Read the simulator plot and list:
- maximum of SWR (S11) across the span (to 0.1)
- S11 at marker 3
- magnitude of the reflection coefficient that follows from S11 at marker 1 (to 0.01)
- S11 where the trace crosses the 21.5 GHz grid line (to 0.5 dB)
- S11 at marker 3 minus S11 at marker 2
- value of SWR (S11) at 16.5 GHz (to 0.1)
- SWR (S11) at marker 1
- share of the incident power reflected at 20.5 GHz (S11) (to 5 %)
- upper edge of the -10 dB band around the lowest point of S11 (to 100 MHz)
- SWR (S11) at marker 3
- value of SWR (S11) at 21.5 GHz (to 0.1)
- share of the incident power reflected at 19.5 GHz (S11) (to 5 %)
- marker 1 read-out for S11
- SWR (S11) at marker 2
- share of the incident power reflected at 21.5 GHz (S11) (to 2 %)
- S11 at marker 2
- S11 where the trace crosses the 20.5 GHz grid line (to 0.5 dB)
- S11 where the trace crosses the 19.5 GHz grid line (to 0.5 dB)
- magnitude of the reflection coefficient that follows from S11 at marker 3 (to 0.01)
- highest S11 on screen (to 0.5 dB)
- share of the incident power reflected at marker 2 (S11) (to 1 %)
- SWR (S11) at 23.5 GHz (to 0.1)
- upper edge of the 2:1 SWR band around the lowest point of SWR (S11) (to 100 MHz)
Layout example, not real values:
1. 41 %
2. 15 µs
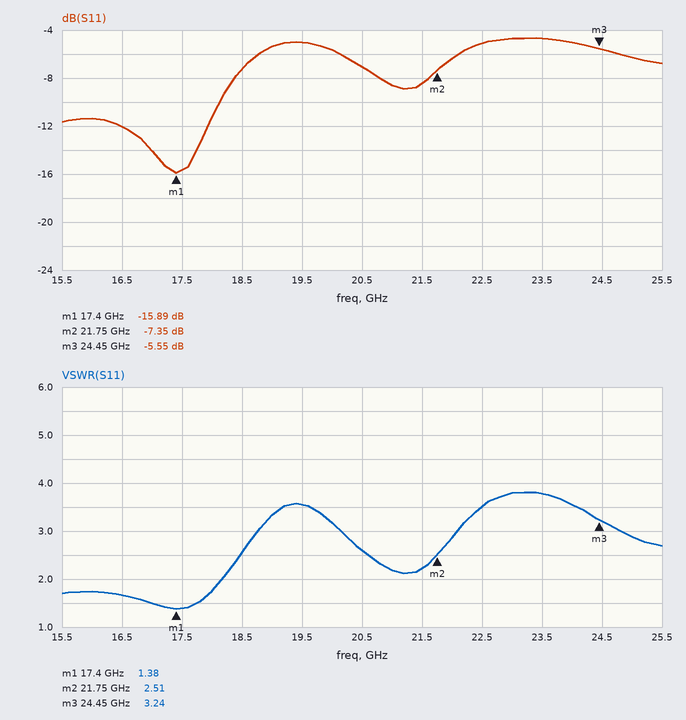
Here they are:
1. 3.8
2. -5.55 dB
3. 0.16
4. -8.5 dB
5. 1.80 dB
6. 1.7
7. 1.38
8. 20 %
9. 18.1 GHz
10. 3.24
11. 2.2
12. 30 %
13. -15.89 dB
14. 2.51
15. 14 %
16. -7.35 dB
17. -7.0 dB
18. -5.0 dB
19. 0.53
20. -4.5 dB
21. 18 %
22. 3.8
23. 18.2 GHz
